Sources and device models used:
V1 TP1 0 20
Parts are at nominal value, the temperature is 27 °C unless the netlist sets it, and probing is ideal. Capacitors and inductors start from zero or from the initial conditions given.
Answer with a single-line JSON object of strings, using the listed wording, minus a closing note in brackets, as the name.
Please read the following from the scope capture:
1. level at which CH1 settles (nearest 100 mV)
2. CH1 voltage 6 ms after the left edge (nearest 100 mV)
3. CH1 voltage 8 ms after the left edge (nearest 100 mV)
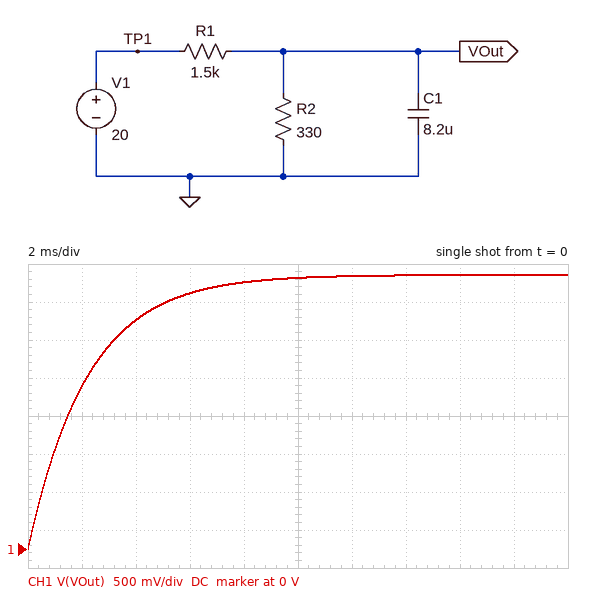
{"level at which CH1 settles": "3.6 V", "CH1 voltage 6 ms after the left edge": "3.4 V", "CH1 voltage 8 ms after the left edge": "3.5 V"}
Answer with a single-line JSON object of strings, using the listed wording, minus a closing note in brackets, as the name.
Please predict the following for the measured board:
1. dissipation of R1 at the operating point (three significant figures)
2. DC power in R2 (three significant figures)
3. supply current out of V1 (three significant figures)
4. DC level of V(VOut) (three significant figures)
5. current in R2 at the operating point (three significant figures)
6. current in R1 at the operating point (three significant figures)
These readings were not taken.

{"dissipation of R1 at the operating point": "179 mW", "DC power in R2": "39.4 mW", "supply current out of V1": "10.9 mA", "DC level of V(VOut)": "3.61 V", "current in R2 at the operating point": "10.9 mA", "current in R1 at the operating point": "10.9 mA"}
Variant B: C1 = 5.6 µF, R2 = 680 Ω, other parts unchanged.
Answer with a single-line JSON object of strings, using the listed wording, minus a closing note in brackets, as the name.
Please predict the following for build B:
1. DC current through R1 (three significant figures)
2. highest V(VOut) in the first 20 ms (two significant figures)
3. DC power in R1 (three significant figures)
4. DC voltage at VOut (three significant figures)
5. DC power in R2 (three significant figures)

{"DC current through R1": "9.17 mA", "highest V(VOut) in the first 20 ms": "6.2 V", "DC power in R1": "126 mW", "DC voltage at VOut": "6.24 V", "DC power in R2": "57.2 mW"}
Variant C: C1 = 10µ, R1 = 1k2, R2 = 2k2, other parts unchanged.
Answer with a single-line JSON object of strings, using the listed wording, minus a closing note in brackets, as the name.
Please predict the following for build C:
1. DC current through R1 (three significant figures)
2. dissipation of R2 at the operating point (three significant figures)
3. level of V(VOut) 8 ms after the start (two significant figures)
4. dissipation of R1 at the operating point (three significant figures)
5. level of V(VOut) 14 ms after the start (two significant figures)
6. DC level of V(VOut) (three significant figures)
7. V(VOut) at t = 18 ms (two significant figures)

{"DC current through R1": "5.88 mA", "dissipation of R2 at the operating point": "76.1 mW", "level of V(VOut) 8 ms after the start": "8.3 V", "dissipation of R1 at the operating point": "41.5 mW", "level of V(VOut) 14 ms after the start": "11 V", "DC level of V(VOut)": "12.9 V", "V(VOut) at t = 18 ms": "12 V"}
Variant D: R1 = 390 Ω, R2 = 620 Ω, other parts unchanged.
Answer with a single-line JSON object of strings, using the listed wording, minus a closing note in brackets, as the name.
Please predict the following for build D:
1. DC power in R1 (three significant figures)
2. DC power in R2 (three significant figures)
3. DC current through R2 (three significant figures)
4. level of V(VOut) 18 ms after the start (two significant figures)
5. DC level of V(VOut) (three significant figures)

{"DC power in R1": "153 mW", "DC power in R2": "243 mW", "DC current through R2": "19.8 mA", "level of V(VOut) 18 ms after the start": "12 V", "DC level of V(VOut)": "12.3 V"}
